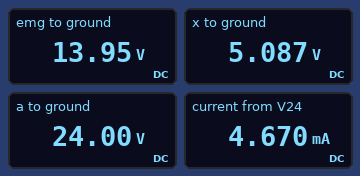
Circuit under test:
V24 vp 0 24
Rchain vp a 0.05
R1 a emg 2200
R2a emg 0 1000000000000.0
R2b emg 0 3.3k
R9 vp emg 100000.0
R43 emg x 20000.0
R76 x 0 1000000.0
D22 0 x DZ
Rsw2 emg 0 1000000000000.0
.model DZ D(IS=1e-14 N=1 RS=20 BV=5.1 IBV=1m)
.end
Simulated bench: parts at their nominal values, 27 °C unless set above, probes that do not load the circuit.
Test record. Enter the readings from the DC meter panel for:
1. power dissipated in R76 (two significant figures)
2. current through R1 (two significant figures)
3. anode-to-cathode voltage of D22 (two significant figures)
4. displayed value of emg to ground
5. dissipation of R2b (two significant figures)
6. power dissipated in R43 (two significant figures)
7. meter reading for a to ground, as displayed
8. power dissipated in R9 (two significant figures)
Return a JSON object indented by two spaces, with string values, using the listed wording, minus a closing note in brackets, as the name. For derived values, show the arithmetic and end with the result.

{
  "power dissipated in R76": "(5.087 V)^2 / 1 MΩ = 26 µW",
  "current through R1": "(24 V - 13.95 V) / 2.2 kΩ = 4.6 mA",
  "anode-to-cathode voltage of D22": "0 V - 5.087 V = -5.1 V",
  "displayed value of emg to ground": "13.95 V",
  "dissipation of R2b": "(13.95 V)^2 / 3.3 kΩ = 59 mW",
  "power dissipated in R43": "(13.95 V - 5.087 V)^2 / 20 kΩ = 3.9 mW",
  "meter reading for a to ground, as displayed": "24.00 V",
  "power dissipated in R9": "(24 V - 13.95 V)^2 / 100 kΩ = 1.0 mW"
}
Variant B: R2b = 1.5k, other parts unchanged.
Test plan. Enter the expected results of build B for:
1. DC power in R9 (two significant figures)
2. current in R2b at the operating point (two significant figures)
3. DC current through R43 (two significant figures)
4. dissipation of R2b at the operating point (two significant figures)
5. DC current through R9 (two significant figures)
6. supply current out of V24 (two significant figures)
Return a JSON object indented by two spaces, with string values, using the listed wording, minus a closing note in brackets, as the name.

{
  "DC power in R9": "2.1 mW",
  "current in R2b at the operating point": "6.4 mA",
  "DC current through R43": "230 µA",
  "dissipation of R2b at the operating point": "62 mW",
  "DC current through R9": "140 µA",
  "supply current out of V24": "6.7 mA"
}
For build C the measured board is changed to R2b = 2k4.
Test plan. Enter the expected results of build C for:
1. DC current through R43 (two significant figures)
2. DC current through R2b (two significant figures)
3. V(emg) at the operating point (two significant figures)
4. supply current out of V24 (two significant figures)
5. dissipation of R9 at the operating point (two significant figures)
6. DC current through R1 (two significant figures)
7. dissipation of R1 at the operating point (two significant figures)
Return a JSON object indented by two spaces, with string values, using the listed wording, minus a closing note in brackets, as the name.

{
  "DC current through R43": "360 µA",
  "DC current through R2b": "5.1 mA",
  "V(emg) at the operating point": "12 V",
  "supply current out of V24": "5.5 mA",
  "dissipation of R9 at the operating point": "1.4 mW",
  "DC current through R1": "5.3 mA",
  "dissipation of R1 at the operating point": "63 mW"
}
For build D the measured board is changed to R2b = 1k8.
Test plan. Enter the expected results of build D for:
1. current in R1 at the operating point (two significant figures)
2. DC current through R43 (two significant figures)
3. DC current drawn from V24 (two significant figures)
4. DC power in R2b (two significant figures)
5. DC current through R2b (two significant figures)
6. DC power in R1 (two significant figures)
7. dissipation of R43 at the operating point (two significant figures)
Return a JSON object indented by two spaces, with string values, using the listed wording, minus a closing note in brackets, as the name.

{
  "current in R1 at the operating point": "6.1 mA",
  "DC current through R43": "280 µA",
  "DC current drawn from V24": "6.2 mA",
  "DC power in R2b": "63 mW",
  "DC current through R2b": "5.9 mA",
  "DC power in R1": "81 mW",
  "dissipation of R43 at the operating point": "1.6 mW"
}
